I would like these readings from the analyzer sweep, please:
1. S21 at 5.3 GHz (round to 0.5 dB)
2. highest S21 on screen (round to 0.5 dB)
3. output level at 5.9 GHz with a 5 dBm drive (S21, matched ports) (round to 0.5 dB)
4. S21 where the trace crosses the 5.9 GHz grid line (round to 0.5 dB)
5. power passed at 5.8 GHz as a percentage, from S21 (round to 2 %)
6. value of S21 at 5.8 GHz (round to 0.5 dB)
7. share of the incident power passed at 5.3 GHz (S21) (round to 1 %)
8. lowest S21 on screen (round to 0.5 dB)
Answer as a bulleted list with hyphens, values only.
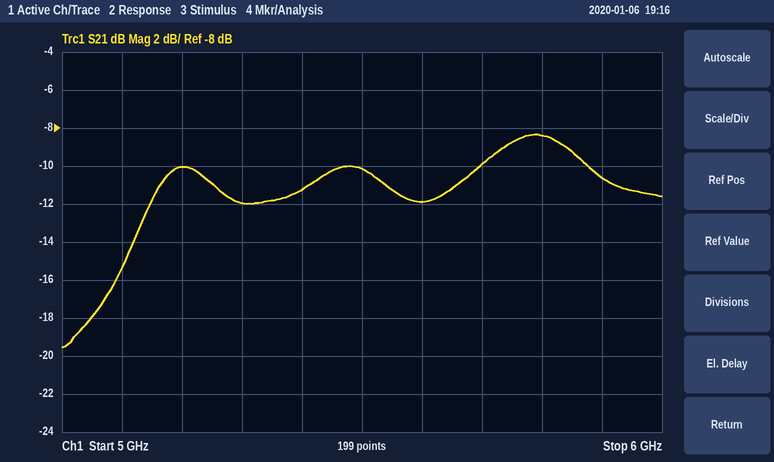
- -12.0 dB
- -8.5 dB
- -5.5 dBm
- -10.5 dB
- 14 %
- -8.5 dB
- 6 %
- -19.5 dB
